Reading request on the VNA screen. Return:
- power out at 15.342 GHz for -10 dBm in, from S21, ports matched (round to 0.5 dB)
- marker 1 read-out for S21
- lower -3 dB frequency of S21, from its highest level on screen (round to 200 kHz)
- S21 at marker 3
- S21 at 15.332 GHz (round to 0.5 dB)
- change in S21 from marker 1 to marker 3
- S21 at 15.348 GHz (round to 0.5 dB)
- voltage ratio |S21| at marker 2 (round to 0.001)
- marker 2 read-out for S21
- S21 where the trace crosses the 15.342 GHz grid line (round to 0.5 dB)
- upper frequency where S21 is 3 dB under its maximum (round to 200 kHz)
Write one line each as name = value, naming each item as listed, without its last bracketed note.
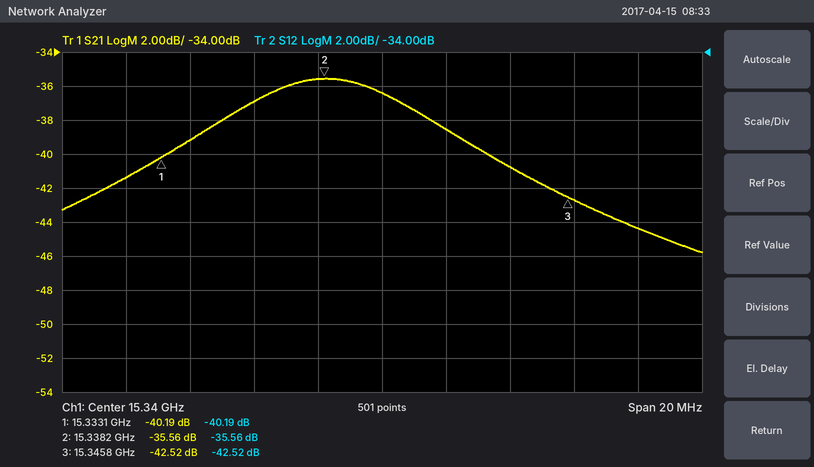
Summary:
power out at 15.342 GHz for -10 dBm in, from S21, ports matched = -48.5 dBm
marker 1 read-out for S21 = -40.19 dB
lower -3 dB frequency of S21, from its highest level on screen = 15.3346 GHz
S21 at marker 3 = -42.52 dB
S21 at 15.332 GHz = -41.5 dB
change in S21 from marker 1 to marker 3 = -2.33 dB
S21 at 15.348 GHz = -44.5 dB
voltage ratio |S21| at marker 2 = 0.017
marker 2 read-out for S21 = -35.56 dB
S21 where the trace crosses the 15.342 GHz grid line = -38.5 dB
upper frequency where S21 is 3 dB under its maximum = 15.3420 GHz
